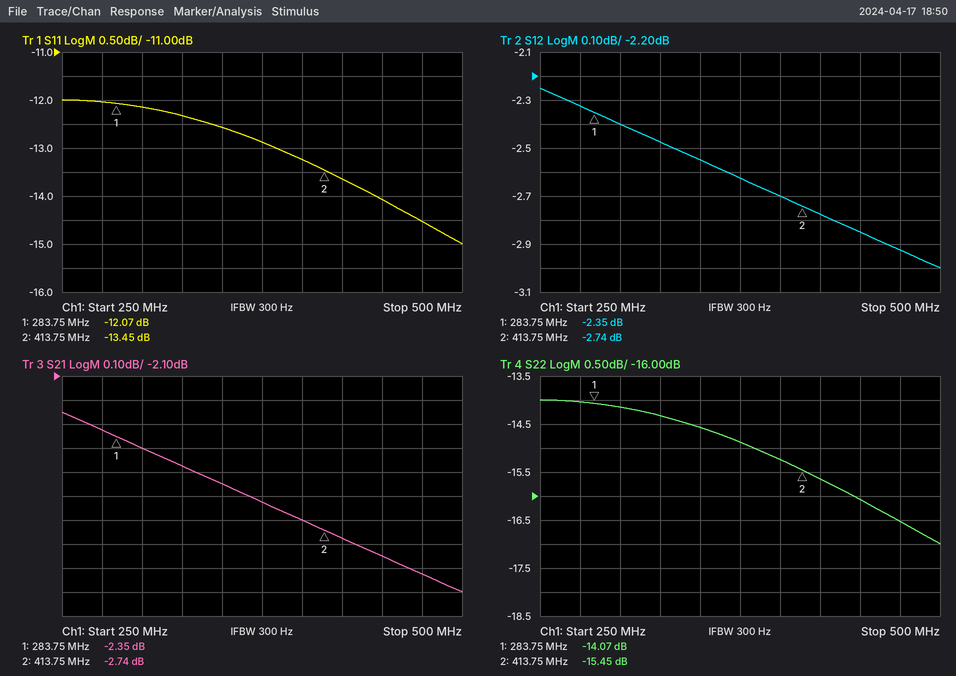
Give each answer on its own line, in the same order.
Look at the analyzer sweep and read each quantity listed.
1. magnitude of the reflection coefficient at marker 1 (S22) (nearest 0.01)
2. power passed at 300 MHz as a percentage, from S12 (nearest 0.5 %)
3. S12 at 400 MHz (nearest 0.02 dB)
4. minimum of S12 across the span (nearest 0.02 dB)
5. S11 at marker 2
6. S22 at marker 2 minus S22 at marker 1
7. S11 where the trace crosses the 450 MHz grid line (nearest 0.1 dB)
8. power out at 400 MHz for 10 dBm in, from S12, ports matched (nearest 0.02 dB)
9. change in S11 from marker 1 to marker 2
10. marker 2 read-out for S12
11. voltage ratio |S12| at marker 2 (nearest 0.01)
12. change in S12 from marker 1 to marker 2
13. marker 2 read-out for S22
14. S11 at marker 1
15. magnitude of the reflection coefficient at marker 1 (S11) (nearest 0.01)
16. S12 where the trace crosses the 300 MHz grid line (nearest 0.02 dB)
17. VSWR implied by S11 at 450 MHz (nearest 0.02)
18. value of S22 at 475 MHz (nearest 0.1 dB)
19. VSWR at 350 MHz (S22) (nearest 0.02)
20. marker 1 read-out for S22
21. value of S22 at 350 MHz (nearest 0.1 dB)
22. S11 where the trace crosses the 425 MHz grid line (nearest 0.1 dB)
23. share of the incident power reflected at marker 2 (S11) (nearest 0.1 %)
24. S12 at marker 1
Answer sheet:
0.20
57.5 %
-2.70 dB
-3.00 dB
-13.45 dB
-1.38 dB
-14.1 dB
7.30 dBm
-1.38 dB
-2.74 dB
0.73
-0.39 dB
-15.45 dB
-12.07 dB
0.25
-2.40 dB
1.50
-16.5 dB
1.46
-14.07 dB
-14.6 dB
-13.6 dB
4.5 %
-2.35 dB
